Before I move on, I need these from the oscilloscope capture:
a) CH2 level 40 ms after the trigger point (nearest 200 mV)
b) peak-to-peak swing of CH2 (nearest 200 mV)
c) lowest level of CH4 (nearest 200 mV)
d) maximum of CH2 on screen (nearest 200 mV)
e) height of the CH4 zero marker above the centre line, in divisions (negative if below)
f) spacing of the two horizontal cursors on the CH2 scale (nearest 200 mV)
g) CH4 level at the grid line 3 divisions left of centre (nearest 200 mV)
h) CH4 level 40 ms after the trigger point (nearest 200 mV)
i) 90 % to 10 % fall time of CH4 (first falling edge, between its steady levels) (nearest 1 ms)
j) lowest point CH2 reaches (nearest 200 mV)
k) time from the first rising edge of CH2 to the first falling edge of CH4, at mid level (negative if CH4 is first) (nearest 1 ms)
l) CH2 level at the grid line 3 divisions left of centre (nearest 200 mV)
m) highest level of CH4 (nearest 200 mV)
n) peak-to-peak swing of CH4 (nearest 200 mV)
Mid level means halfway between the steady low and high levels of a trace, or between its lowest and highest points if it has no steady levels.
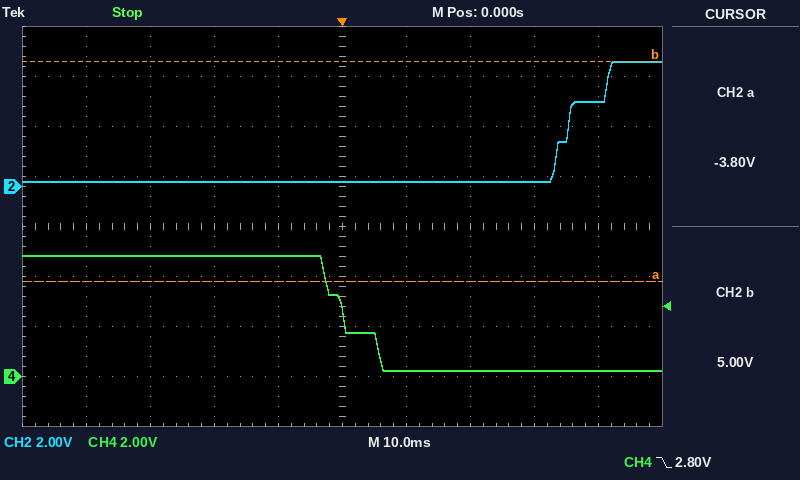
3.4 V
4.8 V
200 mV
5.0 V
-3.0 div
8.8 V
4.8 V
200 mV
9 ms
200 mV
-35 ms
200 mV
4.8 V
4.6 V
